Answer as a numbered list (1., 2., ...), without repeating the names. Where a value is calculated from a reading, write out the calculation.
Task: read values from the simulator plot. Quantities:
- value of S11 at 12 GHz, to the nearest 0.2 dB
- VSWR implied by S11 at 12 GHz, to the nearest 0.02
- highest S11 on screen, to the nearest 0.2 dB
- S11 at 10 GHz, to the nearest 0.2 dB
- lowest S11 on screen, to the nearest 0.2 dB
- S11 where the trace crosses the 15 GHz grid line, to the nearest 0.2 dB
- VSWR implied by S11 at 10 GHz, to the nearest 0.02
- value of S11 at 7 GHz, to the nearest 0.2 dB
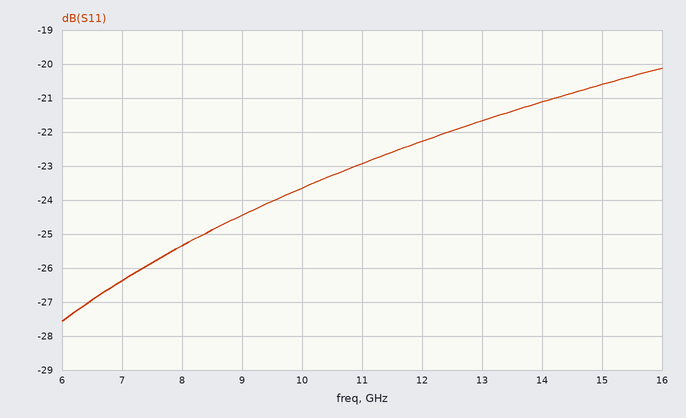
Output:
1. -22.2 dB
2. |Γ| = 10^(-22.2/20) = 0.0776; VSWR = (1 + 0.0776)/(1 − 0.0776) ≈ 1.17, so 1.16 to the nearest 0.02
3. -20.2 dB
4. -23.6 dB
5. -27.6 dB
6. -20.6 dB
7. |Γ| = 10^(-23.6/20) = 0.0661; VSWR = (1 + 0.0661)/(1 − 0.0661) ≈ 1.14
8. -26.4 dB
